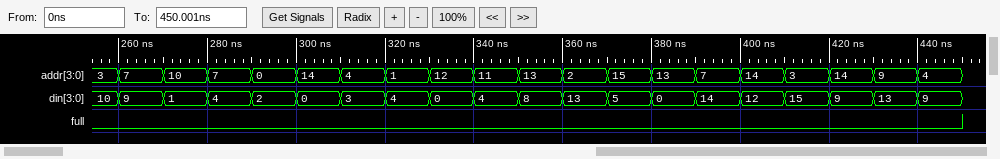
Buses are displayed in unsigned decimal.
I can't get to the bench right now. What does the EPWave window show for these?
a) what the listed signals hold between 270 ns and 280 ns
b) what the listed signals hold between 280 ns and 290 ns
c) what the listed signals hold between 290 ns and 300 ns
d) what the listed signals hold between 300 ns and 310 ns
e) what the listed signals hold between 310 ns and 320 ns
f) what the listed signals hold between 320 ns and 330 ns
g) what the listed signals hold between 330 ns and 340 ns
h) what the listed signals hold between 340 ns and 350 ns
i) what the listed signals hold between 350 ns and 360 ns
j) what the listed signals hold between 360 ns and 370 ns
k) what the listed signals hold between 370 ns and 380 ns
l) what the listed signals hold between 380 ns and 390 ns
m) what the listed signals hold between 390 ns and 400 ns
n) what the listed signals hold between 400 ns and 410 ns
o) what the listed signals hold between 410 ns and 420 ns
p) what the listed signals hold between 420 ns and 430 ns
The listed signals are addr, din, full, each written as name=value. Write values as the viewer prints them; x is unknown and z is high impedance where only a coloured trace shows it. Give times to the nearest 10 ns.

addr=10, din=1, full=0
addr=7, din=4, full=0
addr=0, din=2, full=0
addr=14, din=0, full=0
addr=4, din=3, full=0
addr=1, din=4, full=0
addr=12, din=0, full=0
addr=11, din=4, full=0
addr=13, din=8, full=0
addr=2, din=13, full=0
addr=15, din=5, full=0
addr=13, din=0, full=0
addr=7, din=14, full=0
addr=14, din=12, full=0
addr=3, din=15, full=0
addr=14, din=9, full=0
